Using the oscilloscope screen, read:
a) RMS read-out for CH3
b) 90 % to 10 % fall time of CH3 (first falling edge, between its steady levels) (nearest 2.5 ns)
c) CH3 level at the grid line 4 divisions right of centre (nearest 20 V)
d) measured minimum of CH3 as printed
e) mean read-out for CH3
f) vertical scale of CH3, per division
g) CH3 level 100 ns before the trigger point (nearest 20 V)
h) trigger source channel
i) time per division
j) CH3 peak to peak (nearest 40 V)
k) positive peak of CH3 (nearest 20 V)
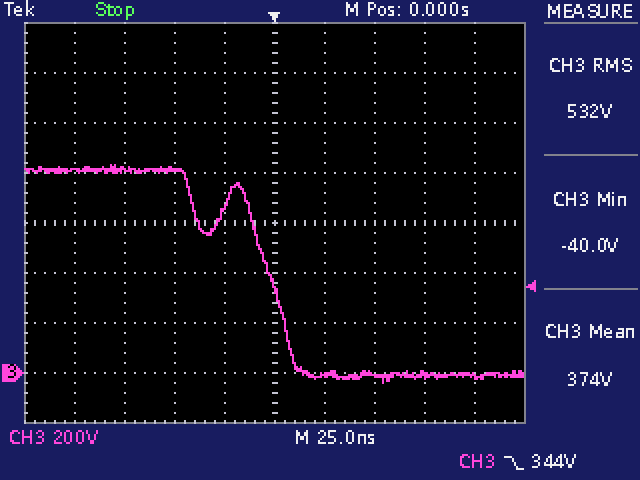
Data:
532 V
25.0 ns
-20 V
-40.0 V
374 V
200 V
820 V
CH3
25 ns
880 V
840 V
